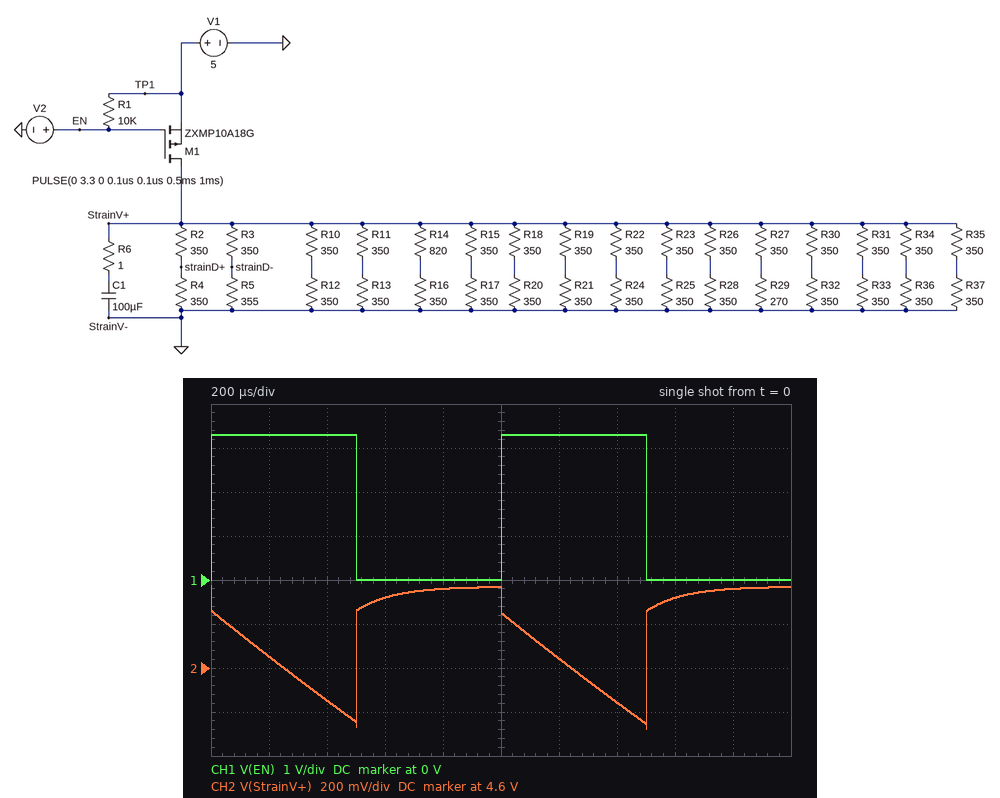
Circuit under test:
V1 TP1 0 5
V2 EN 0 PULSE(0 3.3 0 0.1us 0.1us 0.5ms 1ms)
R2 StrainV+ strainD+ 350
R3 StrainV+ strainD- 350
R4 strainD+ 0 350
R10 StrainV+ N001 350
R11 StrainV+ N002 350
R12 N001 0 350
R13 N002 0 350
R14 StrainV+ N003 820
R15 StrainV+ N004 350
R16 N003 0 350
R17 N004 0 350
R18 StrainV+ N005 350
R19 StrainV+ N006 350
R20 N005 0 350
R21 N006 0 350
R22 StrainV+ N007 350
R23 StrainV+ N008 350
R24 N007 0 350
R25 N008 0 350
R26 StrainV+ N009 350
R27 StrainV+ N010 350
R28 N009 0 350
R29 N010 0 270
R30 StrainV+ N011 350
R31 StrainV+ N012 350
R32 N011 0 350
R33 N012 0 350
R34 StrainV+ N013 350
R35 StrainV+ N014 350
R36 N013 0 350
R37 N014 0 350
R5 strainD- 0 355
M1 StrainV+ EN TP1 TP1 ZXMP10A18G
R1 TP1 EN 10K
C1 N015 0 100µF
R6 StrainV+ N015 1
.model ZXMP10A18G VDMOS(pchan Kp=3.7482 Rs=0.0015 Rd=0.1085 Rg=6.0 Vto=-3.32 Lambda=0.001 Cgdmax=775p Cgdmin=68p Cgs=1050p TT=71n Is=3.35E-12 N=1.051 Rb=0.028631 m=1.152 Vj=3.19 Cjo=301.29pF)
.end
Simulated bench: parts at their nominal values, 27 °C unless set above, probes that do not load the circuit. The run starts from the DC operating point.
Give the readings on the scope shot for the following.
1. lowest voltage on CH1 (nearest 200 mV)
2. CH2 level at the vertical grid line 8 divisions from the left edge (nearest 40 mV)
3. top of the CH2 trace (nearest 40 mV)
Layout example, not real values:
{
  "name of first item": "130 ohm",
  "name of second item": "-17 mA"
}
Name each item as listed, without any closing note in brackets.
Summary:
{
  "lowest voltage on CH1": "0 V",
  "CH2 level at the vertical grid line 8 divisions from the left edge": "4.92 V",
  "top of the CH2 trace": "4.96 V"
}
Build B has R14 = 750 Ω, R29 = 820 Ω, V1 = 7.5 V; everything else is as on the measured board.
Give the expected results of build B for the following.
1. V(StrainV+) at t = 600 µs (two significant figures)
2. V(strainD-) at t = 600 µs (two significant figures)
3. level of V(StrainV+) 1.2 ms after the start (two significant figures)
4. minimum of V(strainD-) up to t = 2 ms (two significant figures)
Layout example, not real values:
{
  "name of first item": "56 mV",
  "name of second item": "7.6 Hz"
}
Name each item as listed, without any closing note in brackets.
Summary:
{
  "V(StrainV+) at t = 600 µs": "7.5 V",
  "V(strainD-) at t = 600 µs": "3.8 V",
  "level of V(StrainV+) 1.2 ms after the start": "7.4 V",
  "minimum of V(strainD-) up to t = 2 ms": "3.7 V"
}
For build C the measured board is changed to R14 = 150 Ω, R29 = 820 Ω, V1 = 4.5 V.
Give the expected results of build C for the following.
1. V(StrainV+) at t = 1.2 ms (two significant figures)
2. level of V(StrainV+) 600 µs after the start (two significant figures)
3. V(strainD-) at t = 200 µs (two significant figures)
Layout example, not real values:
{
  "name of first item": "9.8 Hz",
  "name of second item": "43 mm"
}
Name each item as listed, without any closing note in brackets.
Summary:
{
  "V(StrainV+) at t = 1.2 ms": "4.2 V",
  "level of V(StrainV+) 600 µs after the start": "4.4 V",
  "V(strainD-) at t = 200 µs": "2.1 V"
}
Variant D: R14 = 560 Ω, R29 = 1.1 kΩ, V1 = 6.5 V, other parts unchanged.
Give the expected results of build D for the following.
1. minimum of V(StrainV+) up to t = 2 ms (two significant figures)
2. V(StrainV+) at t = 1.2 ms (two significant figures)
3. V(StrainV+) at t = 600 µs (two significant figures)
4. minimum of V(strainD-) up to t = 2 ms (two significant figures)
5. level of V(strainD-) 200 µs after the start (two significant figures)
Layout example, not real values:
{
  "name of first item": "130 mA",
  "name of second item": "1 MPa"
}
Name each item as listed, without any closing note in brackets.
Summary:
{
  "minimum of V(StrainV+) up to t = 2 ms": "5.7 V",
  "V(StrainV+) at t = 1.2 ms": "6.1 V",
  "V(StrainV+) at t = 600 µs": "6.4 V",
  "minimum of V(strainD-) up to t = 2 ms": "2.9 V",
  "level of V(strainD-) 200 µs after the start": "3.1 V"
}
